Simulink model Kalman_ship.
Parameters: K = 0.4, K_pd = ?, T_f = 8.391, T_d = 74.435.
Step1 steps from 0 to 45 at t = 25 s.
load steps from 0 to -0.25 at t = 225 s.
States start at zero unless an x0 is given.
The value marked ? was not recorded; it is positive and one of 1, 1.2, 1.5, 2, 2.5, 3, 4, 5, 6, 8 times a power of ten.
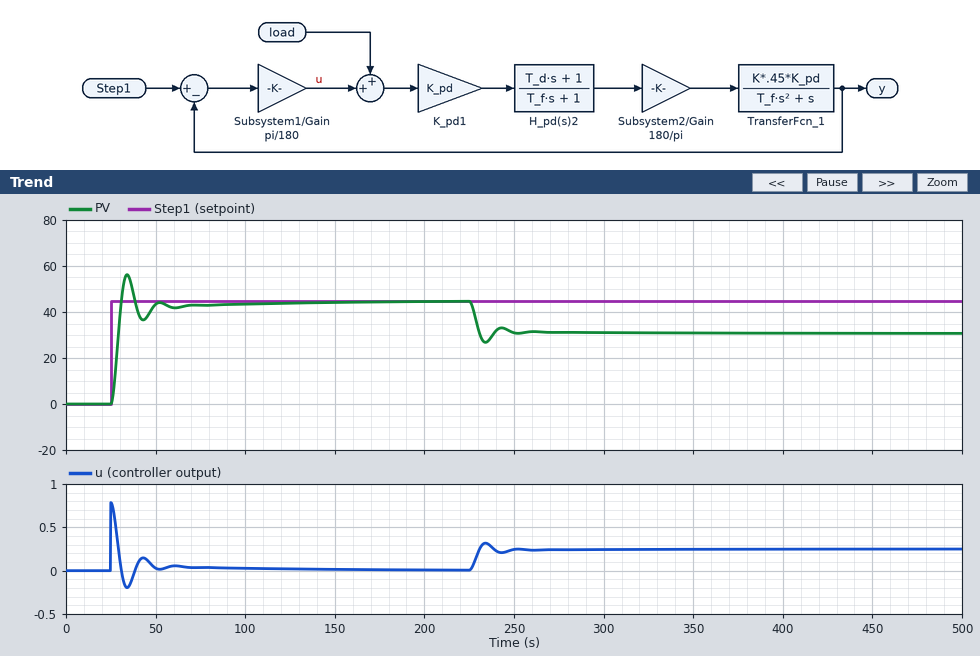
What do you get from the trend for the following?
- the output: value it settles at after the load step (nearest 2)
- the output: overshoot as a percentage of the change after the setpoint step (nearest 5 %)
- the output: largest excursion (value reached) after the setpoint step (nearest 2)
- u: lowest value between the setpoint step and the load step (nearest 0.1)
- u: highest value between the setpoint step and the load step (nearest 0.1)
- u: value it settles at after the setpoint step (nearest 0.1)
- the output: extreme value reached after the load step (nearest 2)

30
25 %
56
-0.2
0.8
0.0
26
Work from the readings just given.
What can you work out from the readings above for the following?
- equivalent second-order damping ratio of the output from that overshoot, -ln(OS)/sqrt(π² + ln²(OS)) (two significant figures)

0.40
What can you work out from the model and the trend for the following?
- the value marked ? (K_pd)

0.8
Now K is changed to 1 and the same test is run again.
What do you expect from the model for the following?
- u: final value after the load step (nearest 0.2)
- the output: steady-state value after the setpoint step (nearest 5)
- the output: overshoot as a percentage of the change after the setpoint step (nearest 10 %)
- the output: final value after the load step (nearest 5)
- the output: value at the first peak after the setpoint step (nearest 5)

0.2
45
50 %
30
65
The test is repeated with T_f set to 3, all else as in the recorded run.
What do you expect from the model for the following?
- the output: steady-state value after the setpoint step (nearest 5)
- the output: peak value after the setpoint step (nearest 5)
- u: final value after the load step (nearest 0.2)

45
55
0.2
